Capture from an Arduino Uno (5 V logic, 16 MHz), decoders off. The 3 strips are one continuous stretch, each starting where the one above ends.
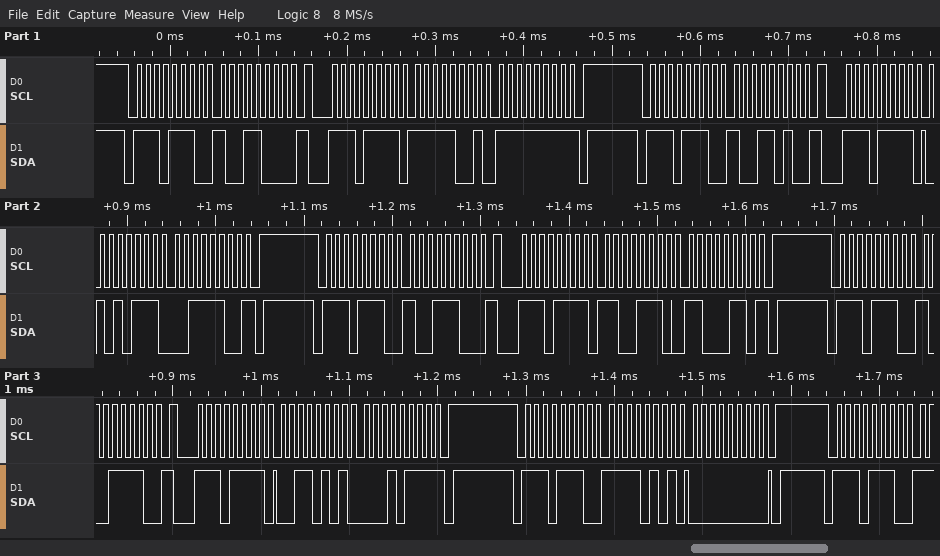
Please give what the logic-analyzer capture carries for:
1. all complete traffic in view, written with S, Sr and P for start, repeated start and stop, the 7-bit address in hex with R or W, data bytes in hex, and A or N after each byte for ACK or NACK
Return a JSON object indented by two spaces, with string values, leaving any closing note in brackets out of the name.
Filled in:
{
  "all complete traffic in view, written with S, Sr and P for start, repeated start and stop, the 7-bit address in hex with R or W, data bytes in hex, and A or N after each byte for ACK or NACK": "S 77W A 98 A Sr 77R A F9 A FF N P S 77W A 9A A Sr 77R A 57 A 3C N P S 77W A 9C A Sr 77R A CE A C6 N P S 77W A 9E A Sr 77R A 35 A 17 N P S 77W A F5 A 00 A P S 77W A"
}
